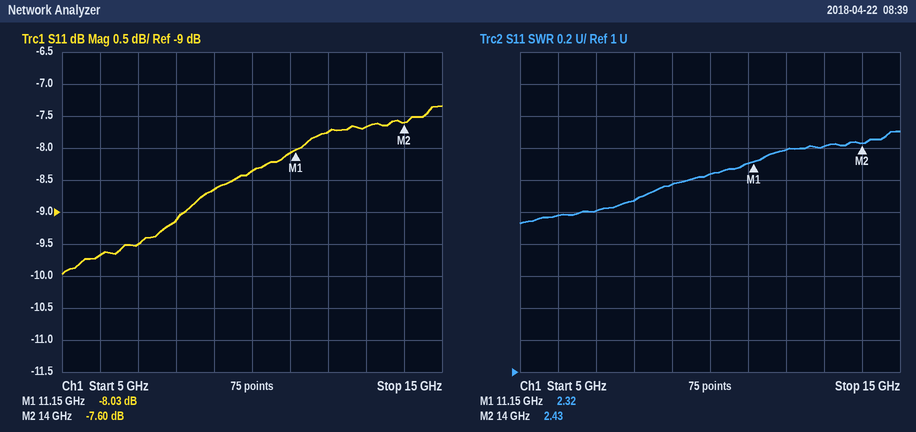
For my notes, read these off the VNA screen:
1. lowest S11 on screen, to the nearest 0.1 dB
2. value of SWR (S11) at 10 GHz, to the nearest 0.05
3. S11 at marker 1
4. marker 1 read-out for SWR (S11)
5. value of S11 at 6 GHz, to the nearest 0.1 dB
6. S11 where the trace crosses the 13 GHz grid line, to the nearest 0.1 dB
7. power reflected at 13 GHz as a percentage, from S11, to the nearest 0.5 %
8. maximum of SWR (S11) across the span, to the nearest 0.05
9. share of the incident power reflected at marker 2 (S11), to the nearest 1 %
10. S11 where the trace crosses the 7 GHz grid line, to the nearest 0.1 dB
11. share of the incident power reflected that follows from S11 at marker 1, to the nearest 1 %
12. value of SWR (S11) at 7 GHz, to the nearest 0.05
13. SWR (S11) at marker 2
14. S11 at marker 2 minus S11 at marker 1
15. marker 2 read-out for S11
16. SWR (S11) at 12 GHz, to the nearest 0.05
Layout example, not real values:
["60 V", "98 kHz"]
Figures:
["-10.0 dB", "2.25", "-8.03 dB", "2.32", "-9.7 dB", "-7.7 dB", "17.0 %", "2.50", "17 %", "-9.5 dB", "16 %", "2.00", "2.43", "0.43 dB", "-7.60 dB", "2.40"]
